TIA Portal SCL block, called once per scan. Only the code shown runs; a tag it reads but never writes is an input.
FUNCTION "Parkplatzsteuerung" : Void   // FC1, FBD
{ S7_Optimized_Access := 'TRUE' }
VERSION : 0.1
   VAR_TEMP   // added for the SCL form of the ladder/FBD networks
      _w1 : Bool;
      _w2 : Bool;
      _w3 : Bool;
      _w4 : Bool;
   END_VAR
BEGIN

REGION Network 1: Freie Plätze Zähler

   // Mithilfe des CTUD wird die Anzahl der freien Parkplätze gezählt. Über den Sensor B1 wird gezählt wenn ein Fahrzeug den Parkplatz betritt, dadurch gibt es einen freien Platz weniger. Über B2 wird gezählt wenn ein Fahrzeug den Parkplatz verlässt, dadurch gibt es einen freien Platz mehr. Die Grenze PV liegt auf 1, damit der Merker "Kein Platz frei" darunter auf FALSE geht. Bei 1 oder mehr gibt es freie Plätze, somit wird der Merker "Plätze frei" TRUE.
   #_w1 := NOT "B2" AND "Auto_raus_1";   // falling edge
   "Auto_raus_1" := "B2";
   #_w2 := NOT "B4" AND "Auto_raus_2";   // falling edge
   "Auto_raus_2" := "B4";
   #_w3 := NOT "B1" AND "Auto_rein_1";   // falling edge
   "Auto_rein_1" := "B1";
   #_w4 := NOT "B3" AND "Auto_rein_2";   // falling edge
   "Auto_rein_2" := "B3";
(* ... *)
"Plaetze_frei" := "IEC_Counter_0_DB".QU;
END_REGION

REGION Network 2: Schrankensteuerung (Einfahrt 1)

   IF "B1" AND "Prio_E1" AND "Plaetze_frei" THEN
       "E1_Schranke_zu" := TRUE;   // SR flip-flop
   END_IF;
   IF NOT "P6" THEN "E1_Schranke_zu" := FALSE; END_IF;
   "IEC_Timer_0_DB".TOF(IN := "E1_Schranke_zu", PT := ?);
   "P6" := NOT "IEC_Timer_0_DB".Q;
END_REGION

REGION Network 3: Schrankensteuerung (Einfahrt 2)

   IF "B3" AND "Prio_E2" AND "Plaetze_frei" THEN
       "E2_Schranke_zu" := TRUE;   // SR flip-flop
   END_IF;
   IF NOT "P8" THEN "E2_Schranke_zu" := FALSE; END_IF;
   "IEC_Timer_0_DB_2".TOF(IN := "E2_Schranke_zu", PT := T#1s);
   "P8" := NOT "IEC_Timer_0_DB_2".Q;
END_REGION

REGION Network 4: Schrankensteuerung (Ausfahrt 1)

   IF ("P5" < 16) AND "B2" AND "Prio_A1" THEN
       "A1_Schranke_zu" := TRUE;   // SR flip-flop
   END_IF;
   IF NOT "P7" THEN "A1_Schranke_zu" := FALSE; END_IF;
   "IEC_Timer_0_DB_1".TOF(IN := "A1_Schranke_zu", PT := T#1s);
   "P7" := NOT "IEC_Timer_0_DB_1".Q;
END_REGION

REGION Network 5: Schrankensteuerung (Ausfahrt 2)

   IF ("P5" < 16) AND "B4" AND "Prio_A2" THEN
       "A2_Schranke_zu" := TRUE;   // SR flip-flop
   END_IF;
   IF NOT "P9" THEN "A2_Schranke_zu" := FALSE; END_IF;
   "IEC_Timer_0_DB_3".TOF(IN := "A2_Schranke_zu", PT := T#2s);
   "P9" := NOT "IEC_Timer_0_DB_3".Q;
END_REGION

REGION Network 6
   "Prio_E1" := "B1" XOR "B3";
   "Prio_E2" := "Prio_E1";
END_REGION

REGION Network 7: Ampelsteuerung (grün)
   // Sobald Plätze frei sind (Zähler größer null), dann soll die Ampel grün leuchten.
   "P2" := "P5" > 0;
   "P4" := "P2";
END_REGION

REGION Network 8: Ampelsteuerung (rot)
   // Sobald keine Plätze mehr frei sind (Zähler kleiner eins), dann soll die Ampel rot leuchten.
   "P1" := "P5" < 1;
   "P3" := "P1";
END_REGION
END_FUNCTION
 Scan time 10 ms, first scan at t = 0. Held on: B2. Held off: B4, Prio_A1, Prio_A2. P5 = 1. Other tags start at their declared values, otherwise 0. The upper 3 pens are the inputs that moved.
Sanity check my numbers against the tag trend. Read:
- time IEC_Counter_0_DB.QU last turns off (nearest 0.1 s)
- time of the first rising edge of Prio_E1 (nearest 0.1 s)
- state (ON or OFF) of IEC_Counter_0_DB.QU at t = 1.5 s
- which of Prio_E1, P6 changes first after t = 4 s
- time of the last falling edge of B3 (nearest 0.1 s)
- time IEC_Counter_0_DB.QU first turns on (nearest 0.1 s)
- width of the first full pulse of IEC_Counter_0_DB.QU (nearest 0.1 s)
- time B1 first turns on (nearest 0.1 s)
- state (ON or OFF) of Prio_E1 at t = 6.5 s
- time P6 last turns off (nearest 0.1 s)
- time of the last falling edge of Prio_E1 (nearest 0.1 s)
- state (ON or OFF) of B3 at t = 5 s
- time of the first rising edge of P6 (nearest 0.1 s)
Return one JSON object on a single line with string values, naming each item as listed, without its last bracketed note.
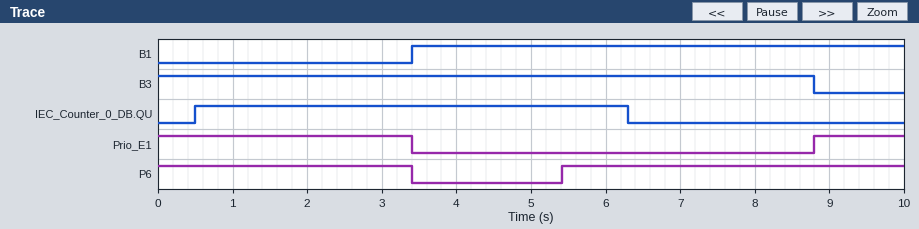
{"time IEC_Counter_0_DB.QU last turns off": "6.3 s", "time of the first rising edge of Prio_E1": "8.8 s", "state (ON or OFF) of IEC_Counter_0_DB.QU at t = 1.5 s": "ON", "which of Prio_E1, P6 changes first after t = 4 s": "P6", "time of the last falling edge of B3": "8.8 s", "time IEC_Counter_0_DB.QU first turns on": "0.5 s", "width of the first full pulse of IEC_Counter_0_DB.QU": "5.8 s", "time B1 first turns on": "3.4 s", "state (ON or OFF) of Prio_E1 at t = 6.5 s": "OFF", "time P6 last turns off": "3.4 s", "time of the last falling edge of Prio_E1": "3.4 s", "state (ON or OFF) of B3 at t = 5 s": "ON", "time of the first rising edge of P6": "5.4 s"}
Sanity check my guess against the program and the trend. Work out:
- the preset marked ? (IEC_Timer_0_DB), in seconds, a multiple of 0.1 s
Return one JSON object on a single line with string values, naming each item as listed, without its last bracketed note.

{"the preset marked ? (IEC_Timer_0_DB), in seconds, a multiple of 0.1 s": "2.0 s"}
